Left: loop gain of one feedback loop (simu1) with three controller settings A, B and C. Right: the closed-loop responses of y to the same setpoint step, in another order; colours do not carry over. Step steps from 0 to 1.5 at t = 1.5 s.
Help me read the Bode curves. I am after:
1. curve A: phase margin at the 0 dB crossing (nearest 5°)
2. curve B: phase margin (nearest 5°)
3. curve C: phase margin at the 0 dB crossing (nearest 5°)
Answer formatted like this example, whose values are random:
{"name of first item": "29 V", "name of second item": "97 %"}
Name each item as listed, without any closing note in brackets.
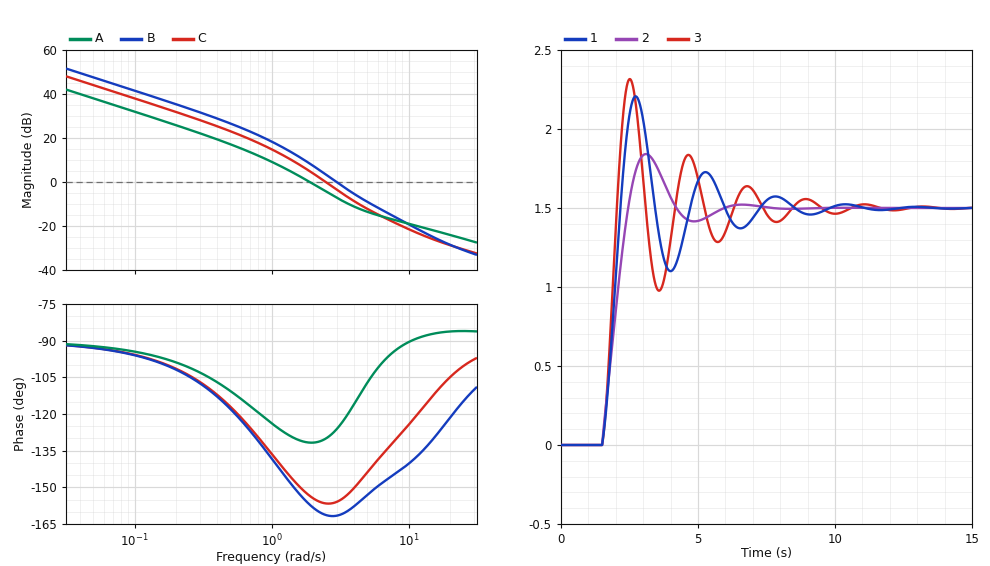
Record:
{"curve A: phase margin at the 0 dB crossing": "50°", "curve B: phase margin": "20°", "curve C: phase margin at the 0 dB crossing": "25°"}
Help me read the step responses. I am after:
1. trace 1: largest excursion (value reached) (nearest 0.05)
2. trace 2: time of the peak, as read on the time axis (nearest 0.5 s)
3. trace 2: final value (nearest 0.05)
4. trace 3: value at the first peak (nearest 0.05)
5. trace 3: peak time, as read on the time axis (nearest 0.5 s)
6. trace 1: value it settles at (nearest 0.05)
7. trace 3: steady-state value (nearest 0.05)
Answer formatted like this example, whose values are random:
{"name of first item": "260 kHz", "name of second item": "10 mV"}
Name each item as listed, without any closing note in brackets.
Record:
{"trace 1: largest excursion (value reached)": "2.20", "trace 2: time of the peak, as read on the time axis": "3.0 s", "trace 2: final value": "1.50", "trace 3: value at the first peak": "2.30", "trace 3: peak time, as read on the time axis": "2.5 s", "trace 1: value it settles at": "1.50", "trace 3: steady-state value": "1.50"}
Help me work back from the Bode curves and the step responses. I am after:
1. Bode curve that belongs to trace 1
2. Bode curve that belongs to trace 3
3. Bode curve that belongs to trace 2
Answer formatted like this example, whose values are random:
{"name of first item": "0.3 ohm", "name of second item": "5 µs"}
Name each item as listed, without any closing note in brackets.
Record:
{"Bode curve that belongs to trace 1": "C", "Bode curve that belongs to trace 3": "B", "Bode curve that belongs to trace 2": "A"}
